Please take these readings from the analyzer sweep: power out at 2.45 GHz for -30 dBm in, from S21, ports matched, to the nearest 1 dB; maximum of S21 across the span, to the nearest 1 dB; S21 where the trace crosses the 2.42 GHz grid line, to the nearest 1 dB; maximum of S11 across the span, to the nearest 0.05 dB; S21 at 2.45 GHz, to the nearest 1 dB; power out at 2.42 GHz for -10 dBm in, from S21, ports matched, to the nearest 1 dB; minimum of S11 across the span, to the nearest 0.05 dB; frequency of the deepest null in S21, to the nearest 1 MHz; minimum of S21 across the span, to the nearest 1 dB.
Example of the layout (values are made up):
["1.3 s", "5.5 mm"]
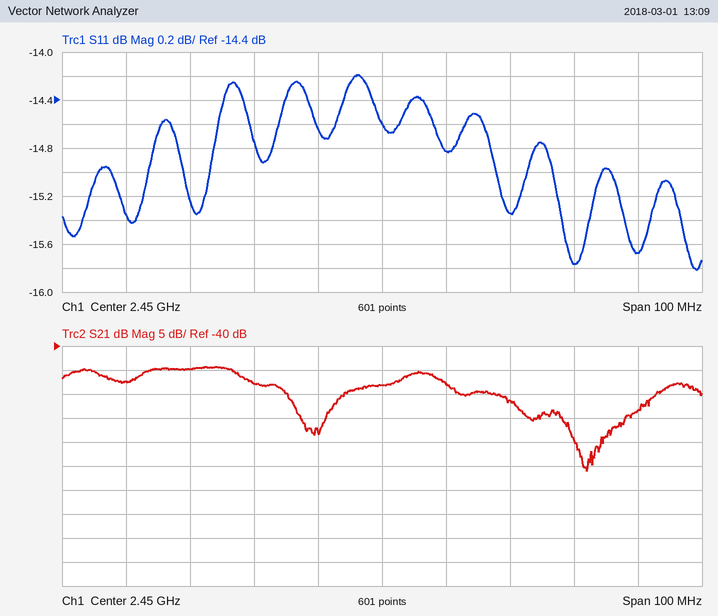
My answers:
["-78 dBm", "-44 dB", "-45 dB", "-14.20 dB", "-48 dB", "-55 dBm", "-15.80 dB", "2.482 GHz", "-66 dB"]
